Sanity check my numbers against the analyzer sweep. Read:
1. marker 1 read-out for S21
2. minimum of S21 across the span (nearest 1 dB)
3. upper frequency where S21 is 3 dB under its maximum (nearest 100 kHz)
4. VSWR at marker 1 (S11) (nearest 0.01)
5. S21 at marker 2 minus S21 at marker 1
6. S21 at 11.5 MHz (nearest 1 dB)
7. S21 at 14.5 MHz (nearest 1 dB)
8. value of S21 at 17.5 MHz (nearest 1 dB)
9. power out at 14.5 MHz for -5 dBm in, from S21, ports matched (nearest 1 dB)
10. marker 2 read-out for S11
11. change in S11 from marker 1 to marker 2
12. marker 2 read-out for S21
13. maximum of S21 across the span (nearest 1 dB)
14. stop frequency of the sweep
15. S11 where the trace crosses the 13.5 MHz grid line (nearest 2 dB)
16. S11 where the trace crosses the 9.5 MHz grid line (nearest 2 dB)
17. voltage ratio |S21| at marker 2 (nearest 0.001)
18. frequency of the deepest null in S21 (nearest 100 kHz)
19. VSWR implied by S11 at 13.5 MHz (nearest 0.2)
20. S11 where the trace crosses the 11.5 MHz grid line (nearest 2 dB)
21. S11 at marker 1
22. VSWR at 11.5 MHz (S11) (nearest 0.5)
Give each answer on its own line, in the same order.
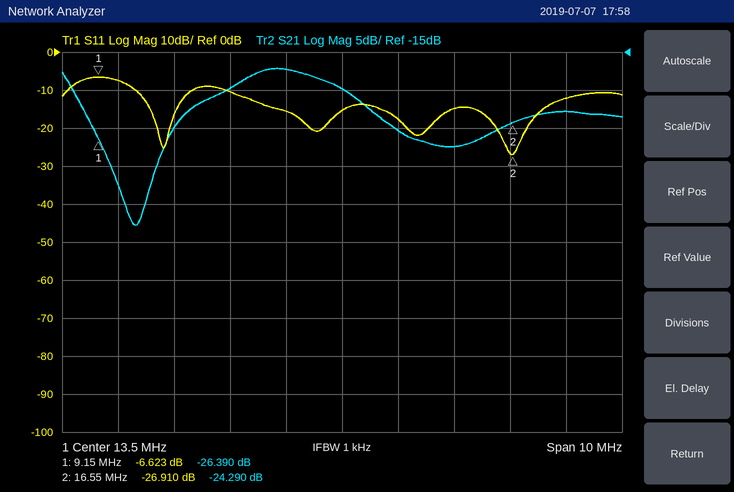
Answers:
-26.390 dB
-38 dB
13.6 MHz
2.75
2.100 dB
-20 dB
-25 dB
-23 dB
-30 dBm
-26.910 dB
-20.287 dB
-24.290 dB
-17 dB
18.5 MHz
-16 dB
-8 dB
0.061
9.8 MHz
1.4
-10 dB
-6.623 dB
2.0
